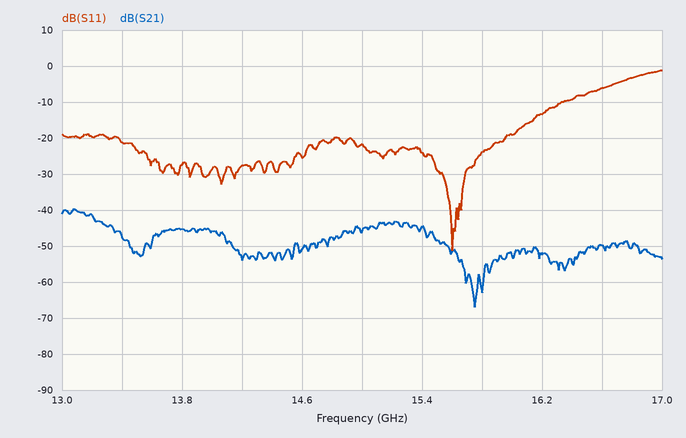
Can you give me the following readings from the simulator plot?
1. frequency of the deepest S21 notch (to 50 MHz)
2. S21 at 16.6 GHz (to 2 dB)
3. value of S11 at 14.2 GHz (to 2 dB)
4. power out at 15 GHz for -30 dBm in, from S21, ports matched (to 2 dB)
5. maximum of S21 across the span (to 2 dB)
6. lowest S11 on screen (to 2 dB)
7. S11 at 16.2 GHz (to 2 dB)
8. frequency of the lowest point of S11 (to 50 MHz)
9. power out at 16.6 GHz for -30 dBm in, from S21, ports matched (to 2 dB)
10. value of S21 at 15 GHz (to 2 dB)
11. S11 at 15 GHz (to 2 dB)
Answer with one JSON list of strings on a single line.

["15.75 GHz", "-50 dB", "-28 dB", "-76 dBm", "-40 dB", "-52 dB", "-14 dB", "15.60 GHz", "-80 dBm", "-46 dB", "-22 dB"]
